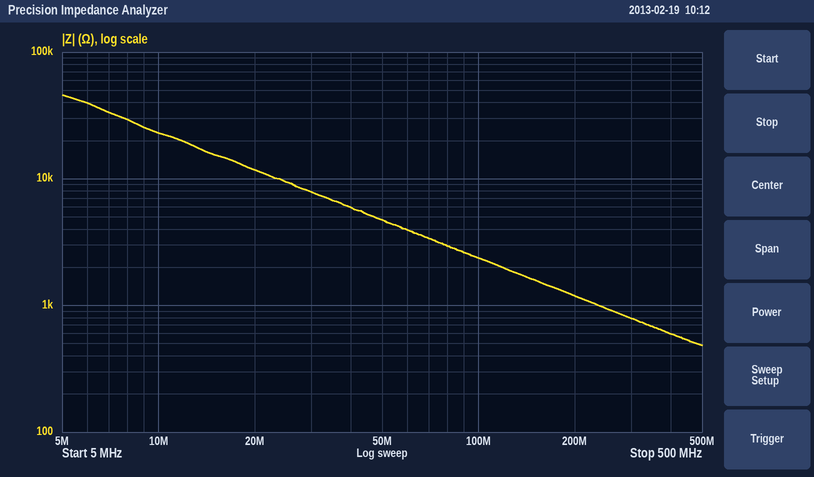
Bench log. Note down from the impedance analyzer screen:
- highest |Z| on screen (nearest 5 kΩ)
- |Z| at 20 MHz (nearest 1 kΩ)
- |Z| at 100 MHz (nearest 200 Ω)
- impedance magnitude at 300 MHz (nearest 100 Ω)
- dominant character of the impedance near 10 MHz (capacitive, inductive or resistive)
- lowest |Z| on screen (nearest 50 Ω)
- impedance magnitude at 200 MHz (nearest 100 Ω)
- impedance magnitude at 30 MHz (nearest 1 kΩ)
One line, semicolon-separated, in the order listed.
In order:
45 kΩ; 12 kΩ; 2.4 kΩ; 800 Ω; capacitive; 500 Ω; 1.2 kΩ; 8 kΩ
